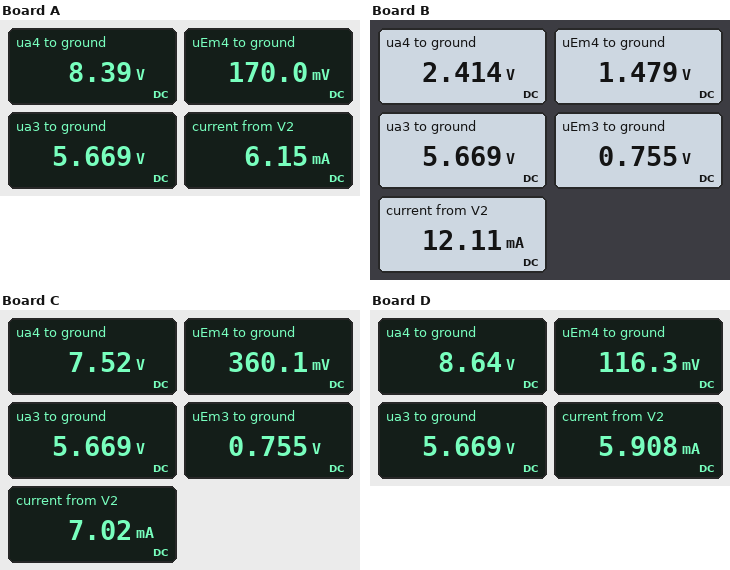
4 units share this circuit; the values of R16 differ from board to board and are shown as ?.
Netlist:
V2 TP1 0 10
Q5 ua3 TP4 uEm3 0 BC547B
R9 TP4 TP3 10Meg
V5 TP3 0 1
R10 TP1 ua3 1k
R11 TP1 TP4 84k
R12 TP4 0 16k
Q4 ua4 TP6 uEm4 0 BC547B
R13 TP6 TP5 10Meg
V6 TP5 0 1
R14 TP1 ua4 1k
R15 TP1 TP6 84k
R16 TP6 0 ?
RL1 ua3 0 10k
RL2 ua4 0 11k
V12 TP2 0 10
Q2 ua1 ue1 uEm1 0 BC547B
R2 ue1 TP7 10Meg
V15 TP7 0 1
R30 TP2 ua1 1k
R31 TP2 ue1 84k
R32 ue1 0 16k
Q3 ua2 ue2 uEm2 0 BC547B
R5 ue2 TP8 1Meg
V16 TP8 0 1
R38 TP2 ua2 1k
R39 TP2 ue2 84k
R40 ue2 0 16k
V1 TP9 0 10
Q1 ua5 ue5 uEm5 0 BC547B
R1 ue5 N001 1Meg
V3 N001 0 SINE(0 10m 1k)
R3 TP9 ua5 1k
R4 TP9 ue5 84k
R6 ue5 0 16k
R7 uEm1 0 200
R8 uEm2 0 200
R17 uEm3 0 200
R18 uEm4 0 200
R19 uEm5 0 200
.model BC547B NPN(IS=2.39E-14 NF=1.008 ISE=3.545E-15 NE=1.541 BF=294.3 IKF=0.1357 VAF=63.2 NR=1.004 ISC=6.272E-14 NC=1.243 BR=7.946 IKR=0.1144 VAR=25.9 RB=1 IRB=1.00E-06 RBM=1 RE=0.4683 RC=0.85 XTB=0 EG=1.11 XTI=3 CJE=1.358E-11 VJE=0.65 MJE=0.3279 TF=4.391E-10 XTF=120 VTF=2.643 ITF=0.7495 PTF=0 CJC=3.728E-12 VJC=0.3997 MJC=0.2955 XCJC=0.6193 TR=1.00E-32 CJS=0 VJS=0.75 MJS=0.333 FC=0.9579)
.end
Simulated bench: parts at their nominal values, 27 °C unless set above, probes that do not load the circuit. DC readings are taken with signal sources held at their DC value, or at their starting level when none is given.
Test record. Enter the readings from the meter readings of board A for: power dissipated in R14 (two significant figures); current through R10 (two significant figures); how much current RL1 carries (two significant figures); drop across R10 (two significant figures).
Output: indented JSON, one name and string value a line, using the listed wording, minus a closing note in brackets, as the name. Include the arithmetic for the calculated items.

{
  "power dissipated in R14": "(10 V - 8.39 V)^2 / 1 kΩ = 2.6 mW",
  "current through R10": "(10 V - 5.669 V) / 1 kΩ = 4.3 mA",
  "how much current RL1 carries": "(5.669 V) / 10 kΩ = 570 µA",
  "drop across R10": "10 V - 5.669 V = 4.3 V"
}
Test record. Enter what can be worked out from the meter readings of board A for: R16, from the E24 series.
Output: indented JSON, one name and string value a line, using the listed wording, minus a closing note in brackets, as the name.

{
  "R16, from the E24 series": "7.5 kΩ"
}
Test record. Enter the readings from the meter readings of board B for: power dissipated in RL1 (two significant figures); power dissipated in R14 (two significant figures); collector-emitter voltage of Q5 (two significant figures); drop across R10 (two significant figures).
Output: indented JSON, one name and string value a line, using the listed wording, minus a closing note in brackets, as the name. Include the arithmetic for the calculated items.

{
  "power dissipated in RL1": "(5.669 V)^2 / 10 kΩ = 3.2 mW",
  "power dissipated in R14": "(10 V - 2.414 V)^2 / 1 kΩ = 58 mW",
  "collector-emitter voltage of Q5": "5.669 V - 755 mV = 4.9 V",
  "drop across R10": "10 V - 5.669 V = 4.3 V"
}
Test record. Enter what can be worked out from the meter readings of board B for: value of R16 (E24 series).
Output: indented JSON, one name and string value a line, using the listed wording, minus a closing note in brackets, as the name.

{
  "value of R16": "33 kΩ"
}
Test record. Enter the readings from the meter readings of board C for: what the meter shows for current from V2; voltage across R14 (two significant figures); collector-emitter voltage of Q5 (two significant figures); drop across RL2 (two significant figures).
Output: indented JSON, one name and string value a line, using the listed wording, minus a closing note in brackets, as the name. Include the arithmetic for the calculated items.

{
  "what the meter shows for current from V2": "7.02 mA",
  "voltage across R14": "10 V - 7.52 V = 2.5 V",
  "collector-emitter voltage of Q5": "5.669 V - 755 mV = 4.9 V",
  "drop across RL2": "7.52 V = 7.5 V"
}
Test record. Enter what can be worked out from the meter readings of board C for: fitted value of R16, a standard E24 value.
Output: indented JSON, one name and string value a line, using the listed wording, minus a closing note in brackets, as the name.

{
  "fitted value of R16, a standard E24 value": "10 kΩ"
}
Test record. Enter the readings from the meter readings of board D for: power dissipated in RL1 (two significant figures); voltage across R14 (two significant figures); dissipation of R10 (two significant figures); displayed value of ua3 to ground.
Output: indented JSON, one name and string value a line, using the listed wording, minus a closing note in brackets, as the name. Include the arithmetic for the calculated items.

{
  "power dissipated in RL1": "(5.669 V)^2 / 10 kΩ = 3.2 mW",
  "voltage across R14": "10 V - 8.64 V = 1.4 V",
  "dissipation of R10": "(10 V - 5.669 V)^2 / 1 kΩ = 19 mW",
  "displayed value of ua3 to ground": "5.669 V"
}
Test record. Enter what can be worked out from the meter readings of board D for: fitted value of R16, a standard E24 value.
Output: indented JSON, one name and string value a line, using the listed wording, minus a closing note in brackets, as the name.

{
  "fitted value of R16, a standard E24 value": "6.8 kΩ"
}
